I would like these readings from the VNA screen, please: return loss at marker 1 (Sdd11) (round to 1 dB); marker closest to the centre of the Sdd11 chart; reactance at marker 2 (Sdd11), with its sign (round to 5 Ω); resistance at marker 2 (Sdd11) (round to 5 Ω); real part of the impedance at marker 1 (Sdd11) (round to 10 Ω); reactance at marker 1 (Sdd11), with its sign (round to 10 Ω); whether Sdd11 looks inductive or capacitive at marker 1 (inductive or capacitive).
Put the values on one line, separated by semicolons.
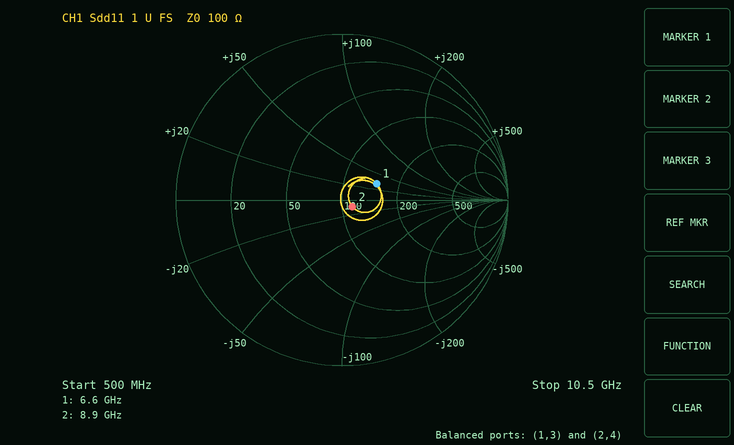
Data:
13 dB; marker 2; -10 Ω; 115 Ω; 150 Ω; +30 Ω; inductive
